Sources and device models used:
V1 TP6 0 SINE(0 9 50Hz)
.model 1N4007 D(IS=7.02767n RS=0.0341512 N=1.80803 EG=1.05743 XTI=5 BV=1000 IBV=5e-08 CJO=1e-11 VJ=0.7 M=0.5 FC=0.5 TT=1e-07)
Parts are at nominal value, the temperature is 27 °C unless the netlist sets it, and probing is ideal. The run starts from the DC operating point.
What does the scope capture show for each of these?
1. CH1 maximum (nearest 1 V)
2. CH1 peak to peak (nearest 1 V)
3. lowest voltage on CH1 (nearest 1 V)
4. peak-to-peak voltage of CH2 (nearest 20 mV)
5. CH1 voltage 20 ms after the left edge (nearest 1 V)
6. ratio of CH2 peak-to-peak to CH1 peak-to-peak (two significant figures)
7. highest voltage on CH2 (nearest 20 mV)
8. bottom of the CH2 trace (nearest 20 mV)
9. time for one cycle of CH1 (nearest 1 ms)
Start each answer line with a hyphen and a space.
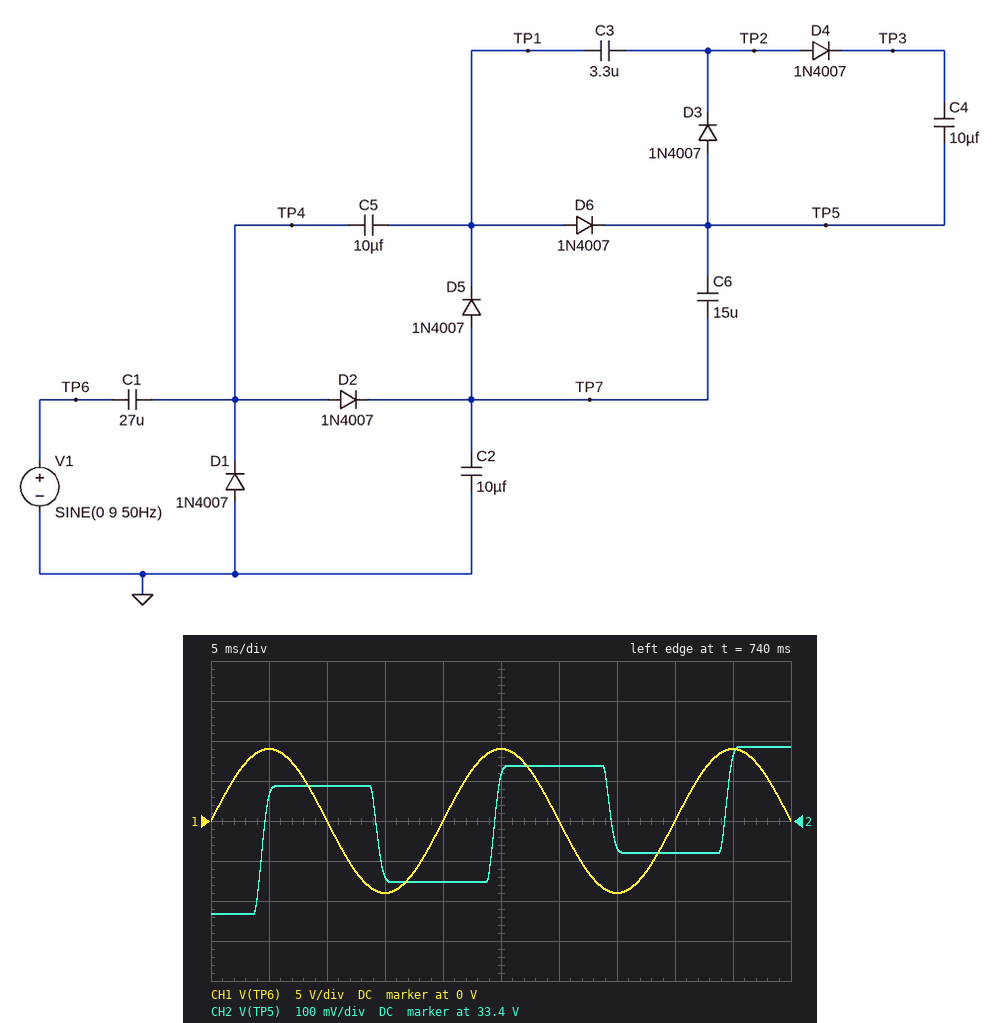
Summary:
- 9 V
- 18 V
- -9 V
- 420 mV
- 0 V
- 0.023
- 33.58 V
- 33.16 V
- 20 ms
